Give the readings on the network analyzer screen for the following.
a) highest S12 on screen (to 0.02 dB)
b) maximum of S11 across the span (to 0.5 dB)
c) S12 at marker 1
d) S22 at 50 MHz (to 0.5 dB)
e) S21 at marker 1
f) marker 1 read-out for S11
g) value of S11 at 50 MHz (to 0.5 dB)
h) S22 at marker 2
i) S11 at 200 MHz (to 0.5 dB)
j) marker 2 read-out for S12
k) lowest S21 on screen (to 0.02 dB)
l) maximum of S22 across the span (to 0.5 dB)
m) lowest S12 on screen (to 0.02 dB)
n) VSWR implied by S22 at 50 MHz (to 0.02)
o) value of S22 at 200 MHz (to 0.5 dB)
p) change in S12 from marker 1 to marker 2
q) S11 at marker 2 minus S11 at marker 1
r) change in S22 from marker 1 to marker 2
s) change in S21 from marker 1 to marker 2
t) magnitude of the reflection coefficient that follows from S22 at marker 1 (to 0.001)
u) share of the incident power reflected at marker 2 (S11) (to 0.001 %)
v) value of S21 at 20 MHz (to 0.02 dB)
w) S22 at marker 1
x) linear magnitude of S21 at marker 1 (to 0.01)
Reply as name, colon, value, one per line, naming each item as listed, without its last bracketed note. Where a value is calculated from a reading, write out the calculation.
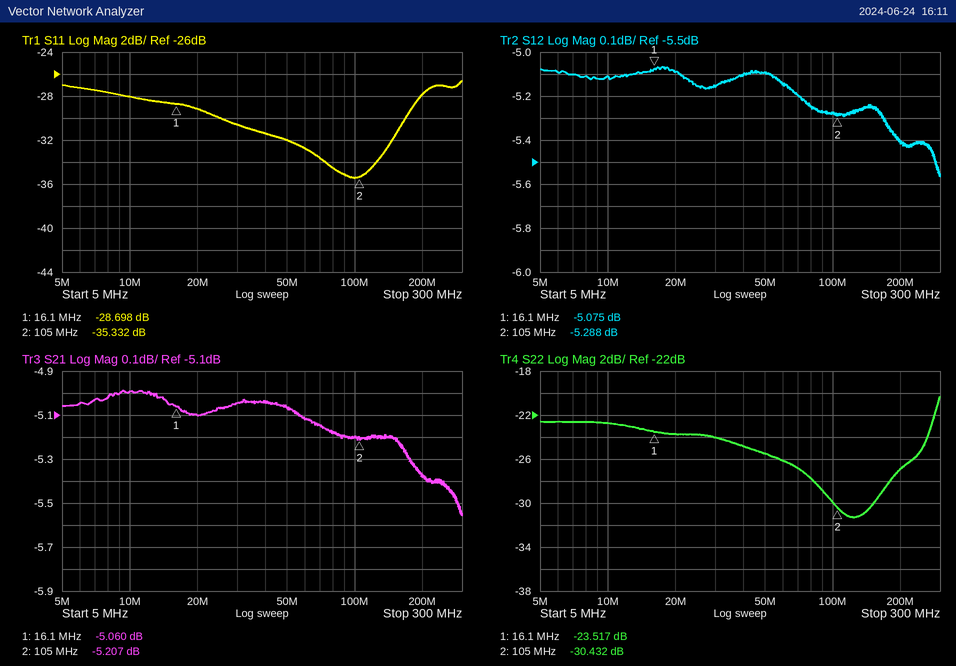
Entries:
highest S12 on screen: -5.06 dB
maximum of S11 across the span: -26.5 dB
S12 at marker 1: -5.075 dB
S22 at 50 MHz: -25.5 dB
S21 at marker 1: -5.060 dB
marker 1 read-out for S11: -28.698 dB
value of S11 at 50 MHz: -32.0 dB
S22 at marker 2: -30.432 dB
S11 at 200 MHz: -28.0 dB
marker 2 read-out for S12: -5.288 dB
lowest S21 on screen: -5.56 dB
maximum of S22 across the span: -20.5 dB
lowest S12 on screen: -5.56 dB
VSWR implied by S22 at 50 MHz: |Γ| = 10^(-25.5/20) = 0.0531; VSWR = (1 + 0.0531)/(1 − 0.0531) ≈ 1.11, so 1.12 to the nearest 0.02
value of S22 at 200 MHz: -27.0 dB
change in S12 from marker 1 to marker 2: -5.288 − (-5.075) = -0.213 dB
S11 at marker 2 minus S11 at marker 1: -35.332 − (-28.698) = -6.634 dB
change in S22 from marker 1 to marker 2: -30.432 − (-23.517) = -6.915 dB
change in S21 from marker 1 to marker 2: -5.207 − (-5.06) = -0.147 dB
magnitude of the reflection coefficient that follows from S22 at marker 1: 10^(-23.517/20) ≈ 0.067
share of the incident power reflected at marker 2 (S11): 10^(-35.332/10) ≈ 0.029 %
value of S21 at 20 MHz: -5.10 dB
S22 at marker 1: -23.517 dB
linear magnitude of S21 at marker 1: 10^(-5.06/20) ≈ 0.56
